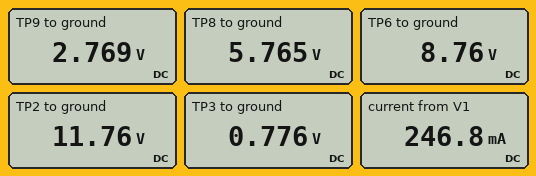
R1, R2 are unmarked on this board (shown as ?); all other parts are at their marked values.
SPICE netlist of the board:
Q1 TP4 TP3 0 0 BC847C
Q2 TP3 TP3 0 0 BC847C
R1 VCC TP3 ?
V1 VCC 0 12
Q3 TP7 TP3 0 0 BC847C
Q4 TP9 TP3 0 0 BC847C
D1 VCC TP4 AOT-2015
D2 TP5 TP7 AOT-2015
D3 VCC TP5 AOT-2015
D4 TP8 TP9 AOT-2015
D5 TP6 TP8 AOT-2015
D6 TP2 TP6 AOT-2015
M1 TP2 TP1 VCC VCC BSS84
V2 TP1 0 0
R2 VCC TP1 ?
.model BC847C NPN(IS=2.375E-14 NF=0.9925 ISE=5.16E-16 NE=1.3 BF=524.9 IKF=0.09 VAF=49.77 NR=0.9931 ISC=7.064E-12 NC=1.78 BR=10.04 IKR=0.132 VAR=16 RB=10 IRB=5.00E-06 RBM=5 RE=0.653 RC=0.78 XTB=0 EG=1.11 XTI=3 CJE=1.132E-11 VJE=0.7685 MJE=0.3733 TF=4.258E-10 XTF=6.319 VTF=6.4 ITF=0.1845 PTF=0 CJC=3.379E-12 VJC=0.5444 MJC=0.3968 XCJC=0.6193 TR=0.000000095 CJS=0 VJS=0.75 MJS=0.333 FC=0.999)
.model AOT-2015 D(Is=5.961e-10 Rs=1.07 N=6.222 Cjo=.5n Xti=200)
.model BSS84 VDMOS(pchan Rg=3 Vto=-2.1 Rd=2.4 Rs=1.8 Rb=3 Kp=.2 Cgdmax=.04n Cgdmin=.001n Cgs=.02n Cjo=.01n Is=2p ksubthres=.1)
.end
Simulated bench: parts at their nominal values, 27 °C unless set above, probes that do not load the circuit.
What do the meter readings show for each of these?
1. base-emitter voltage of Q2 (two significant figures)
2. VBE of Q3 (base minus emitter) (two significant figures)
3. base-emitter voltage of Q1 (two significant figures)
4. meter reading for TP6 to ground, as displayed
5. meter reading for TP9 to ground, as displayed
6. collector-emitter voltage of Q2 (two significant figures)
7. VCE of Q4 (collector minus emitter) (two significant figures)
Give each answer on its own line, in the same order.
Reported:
780 mV
780 mV
780 mV
8.76 V
2.769 V
780 mV
2.8 V
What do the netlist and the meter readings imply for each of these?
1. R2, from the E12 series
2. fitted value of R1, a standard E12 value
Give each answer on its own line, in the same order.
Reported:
330 Ω
220 Ω
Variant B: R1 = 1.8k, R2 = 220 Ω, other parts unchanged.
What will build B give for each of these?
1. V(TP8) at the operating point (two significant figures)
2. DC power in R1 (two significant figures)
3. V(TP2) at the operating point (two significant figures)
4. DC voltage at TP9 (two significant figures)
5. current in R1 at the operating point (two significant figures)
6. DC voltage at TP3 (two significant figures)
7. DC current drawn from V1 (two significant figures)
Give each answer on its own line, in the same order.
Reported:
6.7 V
71 mW
12 V
4.1 V
6.3 mA
680 mV
82 mA
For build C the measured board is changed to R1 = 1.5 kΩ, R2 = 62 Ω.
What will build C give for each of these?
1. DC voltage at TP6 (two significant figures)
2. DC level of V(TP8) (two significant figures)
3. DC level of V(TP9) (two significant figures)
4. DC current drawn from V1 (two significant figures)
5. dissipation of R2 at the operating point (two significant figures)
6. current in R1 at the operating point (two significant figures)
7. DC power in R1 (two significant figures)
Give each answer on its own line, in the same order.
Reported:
9.3 V
6.7 V
4.0 V
230 mA
2.3 W
7.5 mA
85 mW
